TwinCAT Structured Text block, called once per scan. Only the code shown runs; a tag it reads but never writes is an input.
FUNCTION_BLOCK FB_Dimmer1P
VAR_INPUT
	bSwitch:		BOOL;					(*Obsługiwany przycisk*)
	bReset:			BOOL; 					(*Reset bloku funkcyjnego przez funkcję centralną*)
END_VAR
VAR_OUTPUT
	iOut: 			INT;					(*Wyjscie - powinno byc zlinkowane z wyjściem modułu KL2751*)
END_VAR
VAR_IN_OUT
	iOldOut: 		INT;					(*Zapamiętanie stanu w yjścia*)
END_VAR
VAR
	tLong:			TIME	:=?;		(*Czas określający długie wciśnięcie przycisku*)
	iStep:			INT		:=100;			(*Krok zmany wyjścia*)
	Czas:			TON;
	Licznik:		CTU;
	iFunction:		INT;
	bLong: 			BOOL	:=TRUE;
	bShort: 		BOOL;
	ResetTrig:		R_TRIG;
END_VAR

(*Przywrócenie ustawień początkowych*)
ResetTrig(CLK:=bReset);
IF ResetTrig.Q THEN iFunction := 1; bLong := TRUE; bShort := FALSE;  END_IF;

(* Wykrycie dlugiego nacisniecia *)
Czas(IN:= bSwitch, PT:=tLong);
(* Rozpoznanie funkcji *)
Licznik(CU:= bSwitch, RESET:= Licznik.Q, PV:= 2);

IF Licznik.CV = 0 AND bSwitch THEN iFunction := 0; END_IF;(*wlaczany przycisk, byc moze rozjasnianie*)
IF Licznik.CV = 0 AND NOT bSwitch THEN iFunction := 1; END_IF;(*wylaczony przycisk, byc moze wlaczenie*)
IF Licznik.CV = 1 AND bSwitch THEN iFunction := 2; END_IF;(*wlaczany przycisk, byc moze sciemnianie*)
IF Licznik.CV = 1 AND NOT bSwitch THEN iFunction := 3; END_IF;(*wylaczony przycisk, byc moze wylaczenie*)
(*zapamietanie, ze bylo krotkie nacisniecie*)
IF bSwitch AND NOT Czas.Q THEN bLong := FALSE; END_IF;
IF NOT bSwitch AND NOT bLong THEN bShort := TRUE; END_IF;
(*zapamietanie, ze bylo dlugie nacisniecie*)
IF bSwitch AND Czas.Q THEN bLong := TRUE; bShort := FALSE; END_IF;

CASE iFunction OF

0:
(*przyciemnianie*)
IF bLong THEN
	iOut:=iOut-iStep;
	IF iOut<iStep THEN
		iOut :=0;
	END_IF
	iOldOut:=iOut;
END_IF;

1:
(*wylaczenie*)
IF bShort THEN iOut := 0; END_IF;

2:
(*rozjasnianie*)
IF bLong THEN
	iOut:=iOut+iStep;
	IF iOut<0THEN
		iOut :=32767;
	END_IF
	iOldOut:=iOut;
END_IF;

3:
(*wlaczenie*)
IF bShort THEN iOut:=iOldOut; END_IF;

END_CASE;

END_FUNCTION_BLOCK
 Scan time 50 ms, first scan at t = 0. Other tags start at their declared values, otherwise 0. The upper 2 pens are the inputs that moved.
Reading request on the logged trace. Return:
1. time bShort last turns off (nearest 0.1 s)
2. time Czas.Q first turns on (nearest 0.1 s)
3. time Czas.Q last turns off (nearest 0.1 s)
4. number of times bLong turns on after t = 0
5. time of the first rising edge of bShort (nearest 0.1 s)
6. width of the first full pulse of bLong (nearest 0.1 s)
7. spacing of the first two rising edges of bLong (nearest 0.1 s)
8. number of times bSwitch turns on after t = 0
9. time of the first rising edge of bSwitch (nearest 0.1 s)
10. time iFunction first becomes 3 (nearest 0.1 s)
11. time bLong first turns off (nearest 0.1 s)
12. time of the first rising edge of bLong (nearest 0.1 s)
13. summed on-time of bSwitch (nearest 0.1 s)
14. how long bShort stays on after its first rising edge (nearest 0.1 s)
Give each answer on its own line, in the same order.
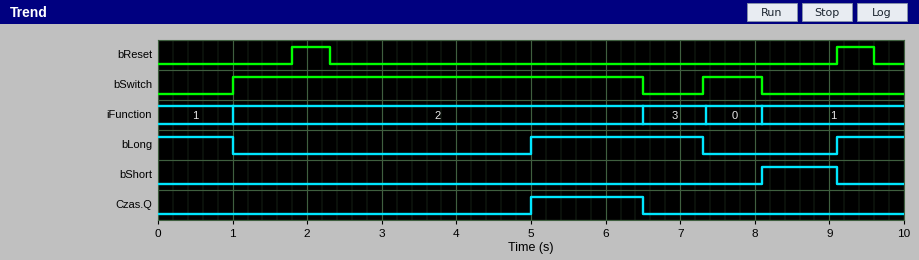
9.1 s
5.0 s
6.5 s
2
8.1 s
2.3 s
4.1 s
2
1.0 s
6.5 s
1.0 s
5.0 s
6.3 s
1.0 s
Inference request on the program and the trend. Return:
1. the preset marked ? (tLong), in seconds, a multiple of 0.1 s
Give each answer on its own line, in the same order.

4.0 s
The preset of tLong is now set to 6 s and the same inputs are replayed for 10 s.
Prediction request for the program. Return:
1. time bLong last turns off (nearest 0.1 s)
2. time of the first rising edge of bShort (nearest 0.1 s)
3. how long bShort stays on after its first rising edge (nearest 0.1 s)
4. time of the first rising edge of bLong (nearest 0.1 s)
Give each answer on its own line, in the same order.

1.0 s
6.5 s
2.6 s
9.1 s
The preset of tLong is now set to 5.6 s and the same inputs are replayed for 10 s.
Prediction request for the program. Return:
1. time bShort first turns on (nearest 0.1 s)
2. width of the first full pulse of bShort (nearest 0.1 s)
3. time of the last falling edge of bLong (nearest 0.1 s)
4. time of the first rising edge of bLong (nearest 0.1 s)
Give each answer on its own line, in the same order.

6.5 s
2.6 s
1.0 s
9.1 s
